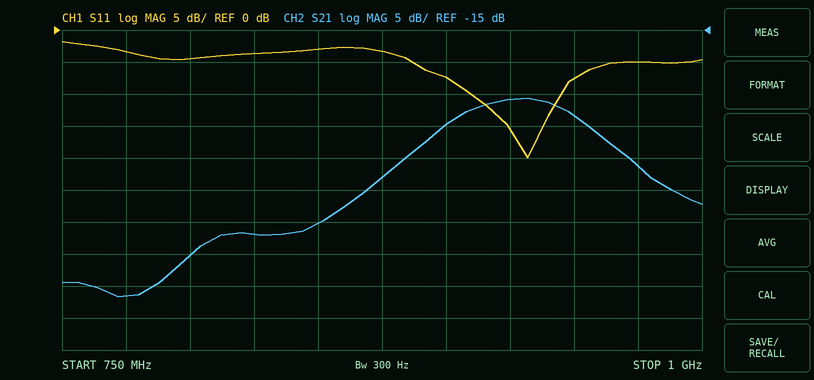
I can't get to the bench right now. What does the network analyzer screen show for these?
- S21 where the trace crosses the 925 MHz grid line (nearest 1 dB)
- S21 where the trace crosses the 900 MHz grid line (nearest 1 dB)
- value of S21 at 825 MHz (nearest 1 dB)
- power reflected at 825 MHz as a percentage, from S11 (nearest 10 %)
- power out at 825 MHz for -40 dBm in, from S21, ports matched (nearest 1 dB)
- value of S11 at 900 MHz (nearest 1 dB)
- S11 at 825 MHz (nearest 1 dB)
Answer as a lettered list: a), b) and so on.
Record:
a) -26 dB
b) -30 dB
c) -47 dB
d) 40 %
e) -87 dBm
f) -7 dB
g) -4 dB
